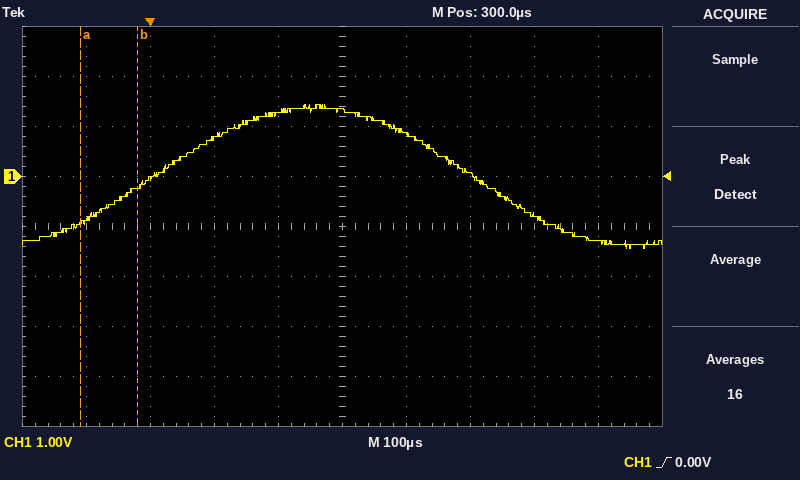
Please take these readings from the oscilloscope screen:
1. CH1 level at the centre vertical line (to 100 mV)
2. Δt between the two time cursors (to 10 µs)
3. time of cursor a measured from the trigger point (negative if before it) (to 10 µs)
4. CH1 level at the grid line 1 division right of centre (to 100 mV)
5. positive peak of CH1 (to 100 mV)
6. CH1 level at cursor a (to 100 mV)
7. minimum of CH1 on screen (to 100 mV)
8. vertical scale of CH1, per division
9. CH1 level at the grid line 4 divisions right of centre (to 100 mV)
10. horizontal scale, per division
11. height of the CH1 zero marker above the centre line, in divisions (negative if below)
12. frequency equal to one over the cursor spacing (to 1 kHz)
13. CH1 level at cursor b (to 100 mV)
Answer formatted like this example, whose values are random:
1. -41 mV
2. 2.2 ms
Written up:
1. 1.3 V
2. 90 µs
3. -110 µs
4. 800 mV
5. 1.4 V
6. -900 mV
7. -1.4 V
8. 1 V
9. -1.3 V
10. 100 µs
11. +1.0 div
12. 11 kHz
13. -200 mV
